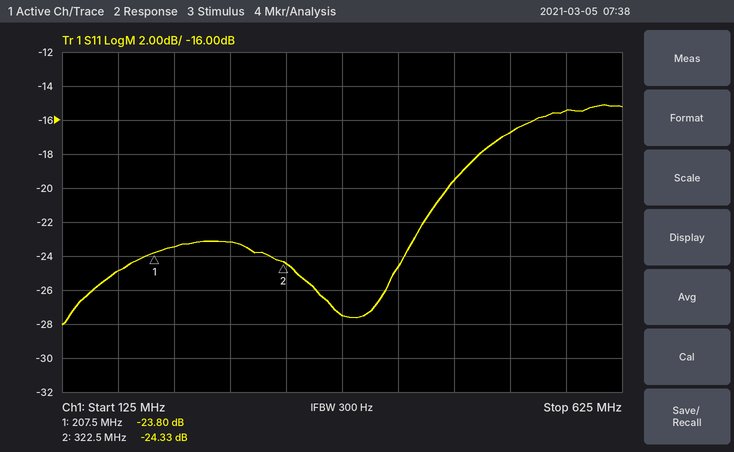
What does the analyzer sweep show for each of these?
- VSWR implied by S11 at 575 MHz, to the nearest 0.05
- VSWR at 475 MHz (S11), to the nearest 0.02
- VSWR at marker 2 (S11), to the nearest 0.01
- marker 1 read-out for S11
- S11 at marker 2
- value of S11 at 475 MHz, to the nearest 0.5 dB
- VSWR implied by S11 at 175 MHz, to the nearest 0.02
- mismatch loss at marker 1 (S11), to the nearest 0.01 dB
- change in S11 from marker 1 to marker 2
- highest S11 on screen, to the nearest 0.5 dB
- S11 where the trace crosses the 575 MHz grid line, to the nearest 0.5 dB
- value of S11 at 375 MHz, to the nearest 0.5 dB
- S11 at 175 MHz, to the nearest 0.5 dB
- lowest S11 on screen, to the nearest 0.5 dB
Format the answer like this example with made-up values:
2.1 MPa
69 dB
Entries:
1.40
1.24
1.13
-23.80 dB
-24.33 dB
-19.5 dB
1.12
0.02 dB
-0.53 dB
-15.0 dB
-15.5 dB
-27.5 dB
-25.0 dB
-28.0 dB
